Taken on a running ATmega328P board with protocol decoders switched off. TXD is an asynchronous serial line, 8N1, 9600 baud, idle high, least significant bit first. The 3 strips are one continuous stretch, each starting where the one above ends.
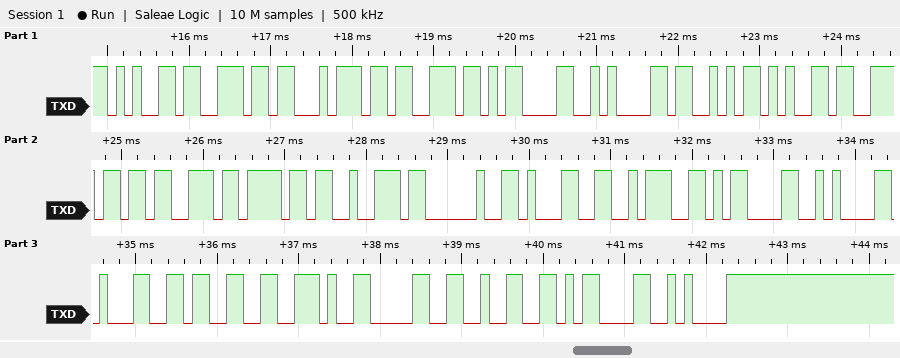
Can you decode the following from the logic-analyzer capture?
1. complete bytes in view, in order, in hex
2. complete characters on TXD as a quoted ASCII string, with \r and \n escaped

0x65 0x6E 0x74 0x73 0x0D 0x0A 0x53 0x65 0x6E 0x73 0x6F 0x72 0x20 0x31 0x3A 0x0D 0x0A 0x31 0x33 0x2E 0x30 0x32 0x0D 0x0A
"ents\r\nSensor 1:\r\n13.02\r\n"
